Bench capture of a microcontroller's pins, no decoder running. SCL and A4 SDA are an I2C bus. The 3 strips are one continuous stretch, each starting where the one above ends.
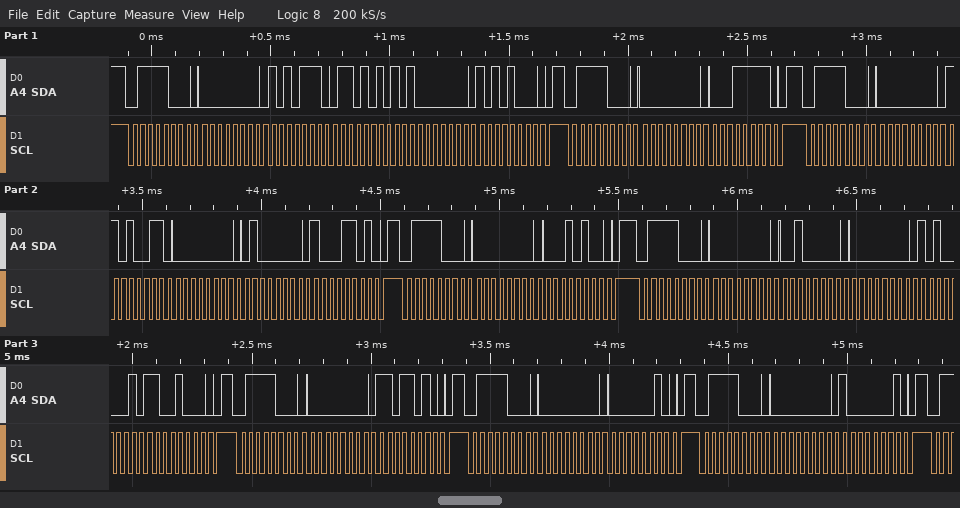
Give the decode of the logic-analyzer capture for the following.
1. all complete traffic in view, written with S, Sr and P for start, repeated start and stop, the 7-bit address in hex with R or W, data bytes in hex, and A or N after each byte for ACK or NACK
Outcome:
S 3CW A 00 A AE A D5 A 80 A A8 A P S 3CW A 00 A 1F A P S 3CW A 00 A D3 A 00 A 40 A 8D A P S 3CW A 00 A 14 A P S 3CW A 00 A 20 A 00 A A1 A C8 A P S 3CW A 00 A DA A P S 3CW A 00 A 02 A P S 3CW A 00 A 81 A P
